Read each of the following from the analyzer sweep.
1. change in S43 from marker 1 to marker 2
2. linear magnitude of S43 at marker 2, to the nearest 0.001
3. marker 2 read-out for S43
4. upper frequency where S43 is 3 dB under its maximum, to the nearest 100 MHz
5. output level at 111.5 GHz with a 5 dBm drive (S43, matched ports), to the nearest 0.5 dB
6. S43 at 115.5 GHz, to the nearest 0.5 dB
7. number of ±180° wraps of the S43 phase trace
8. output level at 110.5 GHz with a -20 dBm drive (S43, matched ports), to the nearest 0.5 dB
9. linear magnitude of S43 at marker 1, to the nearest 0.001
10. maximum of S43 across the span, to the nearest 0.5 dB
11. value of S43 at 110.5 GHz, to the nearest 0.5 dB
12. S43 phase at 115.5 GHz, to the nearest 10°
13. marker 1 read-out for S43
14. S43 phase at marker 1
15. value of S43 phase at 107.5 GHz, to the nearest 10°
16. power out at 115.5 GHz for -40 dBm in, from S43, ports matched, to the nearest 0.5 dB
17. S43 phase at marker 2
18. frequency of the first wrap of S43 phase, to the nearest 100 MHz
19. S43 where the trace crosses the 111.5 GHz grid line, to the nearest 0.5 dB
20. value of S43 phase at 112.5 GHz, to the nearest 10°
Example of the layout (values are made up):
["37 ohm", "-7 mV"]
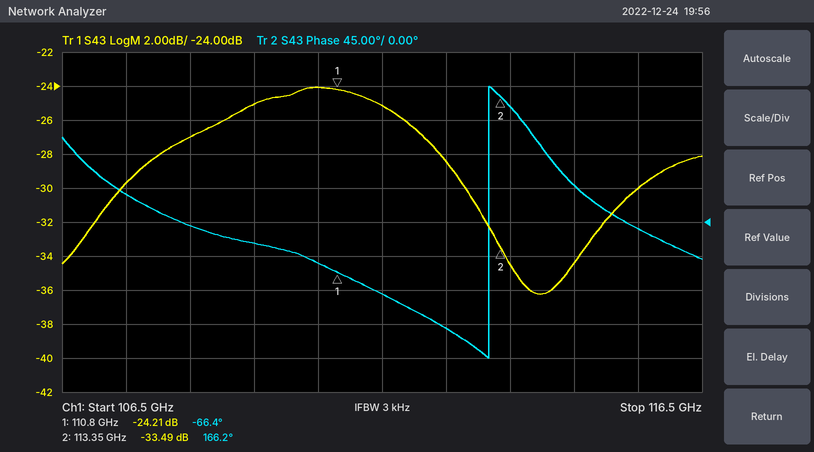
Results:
["-9.28 dB", "0.021", "-33.49 dB", "112.2 GHz", "-20.0 dBm", "-30.0 dB", "1", "-44.0 dBm", "0.062", "-24.0 dB", "-24.0 dB", "-10°", "-24.21 dB", "-66.4°", "40°", "-70.0 dBm", "166.2°", "113.2 GHz", "-25.0 dB", "-140°"]
